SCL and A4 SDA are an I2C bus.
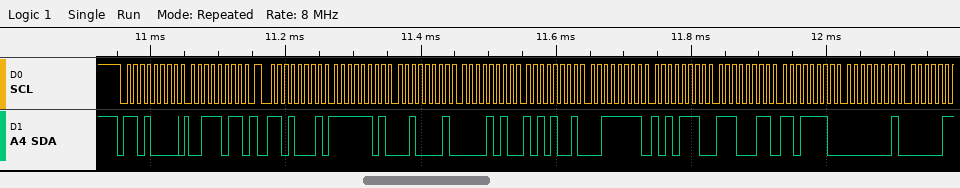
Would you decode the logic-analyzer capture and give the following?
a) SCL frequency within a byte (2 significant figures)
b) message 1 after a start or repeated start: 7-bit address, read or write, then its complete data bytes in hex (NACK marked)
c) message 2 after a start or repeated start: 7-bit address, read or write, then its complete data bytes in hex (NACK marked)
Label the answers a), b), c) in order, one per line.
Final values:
a) 100 kHz
b) 0x68 write: 3B
c) 0x68 read: FD 21 0A A9 3F AE E3 DE 01
